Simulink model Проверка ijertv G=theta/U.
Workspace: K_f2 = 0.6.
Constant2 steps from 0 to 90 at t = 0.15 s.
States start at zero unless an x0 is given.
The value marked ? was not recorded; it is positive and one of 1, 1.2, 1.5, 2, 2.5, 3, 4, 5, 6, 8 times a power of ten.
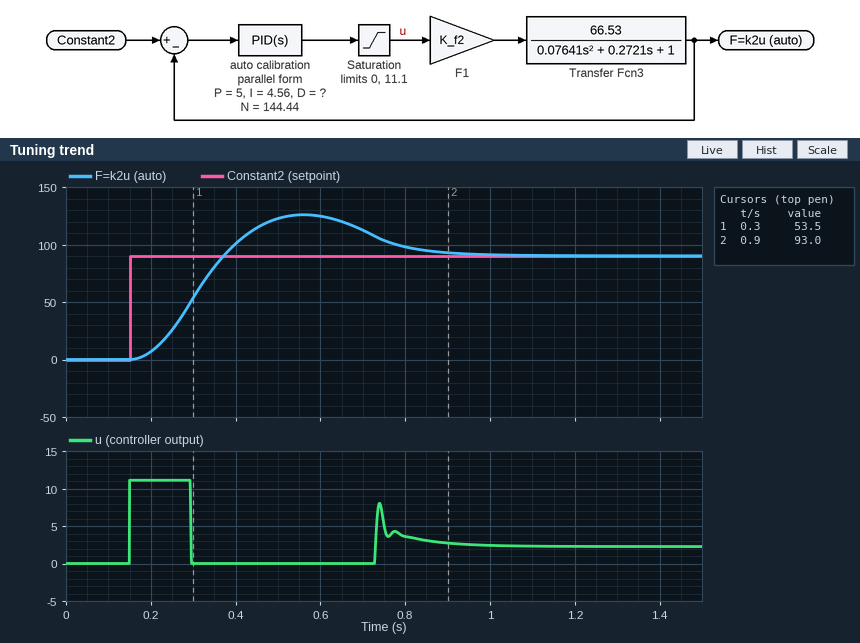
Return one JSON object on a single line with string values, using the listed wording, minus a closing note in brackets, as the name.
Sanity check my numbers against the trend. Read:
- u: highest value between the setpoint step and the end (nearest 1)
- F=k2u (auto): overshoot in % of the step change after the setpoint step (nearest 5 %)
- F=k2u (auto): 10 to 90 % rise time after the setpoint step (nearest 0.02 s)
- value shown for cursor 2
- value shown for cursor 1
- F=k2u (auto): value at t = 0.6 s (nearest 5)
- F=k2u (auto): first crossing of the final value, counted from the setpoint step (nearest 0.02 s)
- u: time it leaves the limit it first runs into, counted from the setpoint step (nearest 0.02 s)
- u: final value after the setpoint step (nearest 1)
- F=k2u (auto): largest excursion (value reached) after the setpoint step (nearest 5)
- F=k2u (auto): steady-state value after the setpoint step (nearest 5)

{"u: highest value between the setpoint step and the end": "11", "F=k2u (auto): overshoot in % of the step change after the setpoint step": "40 %", "F=k2u (auto): 10 to 90 % rise time after the setpoint step": "0.14 s", "value shown for cursor 2": "93.0", "value shown for cursor 1": "53.5", "F=k2u (auto): value at t = 0.6 s": "125", "F=k2u (auto): first crossing of the final value, counted from the setpoint step": "0.22 s", "u: time it leaves the limit it first runs into, counted from the setpoint step": "0.14 s", "u: final value after the setpoint step": "2", "F=k2u (auto): largest excursion (value reached) after the setpoint step": "125", "F=k2u (auto): steady-state value after the setpoint step": "90"}
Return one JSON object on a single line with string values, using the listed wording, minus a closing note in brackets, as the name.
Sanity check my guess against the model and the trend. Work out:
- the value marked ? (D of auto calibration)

{"the value marked ?": "0.4"}
